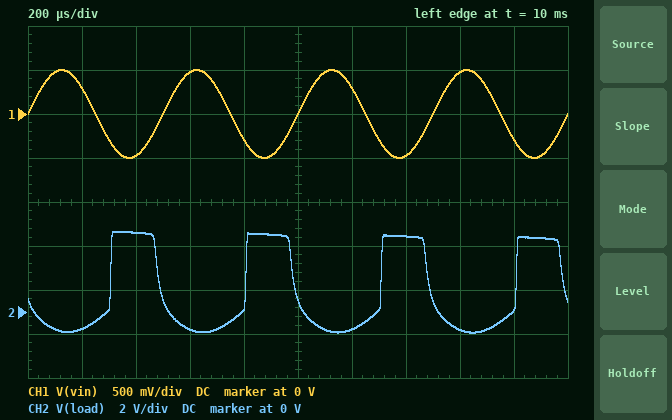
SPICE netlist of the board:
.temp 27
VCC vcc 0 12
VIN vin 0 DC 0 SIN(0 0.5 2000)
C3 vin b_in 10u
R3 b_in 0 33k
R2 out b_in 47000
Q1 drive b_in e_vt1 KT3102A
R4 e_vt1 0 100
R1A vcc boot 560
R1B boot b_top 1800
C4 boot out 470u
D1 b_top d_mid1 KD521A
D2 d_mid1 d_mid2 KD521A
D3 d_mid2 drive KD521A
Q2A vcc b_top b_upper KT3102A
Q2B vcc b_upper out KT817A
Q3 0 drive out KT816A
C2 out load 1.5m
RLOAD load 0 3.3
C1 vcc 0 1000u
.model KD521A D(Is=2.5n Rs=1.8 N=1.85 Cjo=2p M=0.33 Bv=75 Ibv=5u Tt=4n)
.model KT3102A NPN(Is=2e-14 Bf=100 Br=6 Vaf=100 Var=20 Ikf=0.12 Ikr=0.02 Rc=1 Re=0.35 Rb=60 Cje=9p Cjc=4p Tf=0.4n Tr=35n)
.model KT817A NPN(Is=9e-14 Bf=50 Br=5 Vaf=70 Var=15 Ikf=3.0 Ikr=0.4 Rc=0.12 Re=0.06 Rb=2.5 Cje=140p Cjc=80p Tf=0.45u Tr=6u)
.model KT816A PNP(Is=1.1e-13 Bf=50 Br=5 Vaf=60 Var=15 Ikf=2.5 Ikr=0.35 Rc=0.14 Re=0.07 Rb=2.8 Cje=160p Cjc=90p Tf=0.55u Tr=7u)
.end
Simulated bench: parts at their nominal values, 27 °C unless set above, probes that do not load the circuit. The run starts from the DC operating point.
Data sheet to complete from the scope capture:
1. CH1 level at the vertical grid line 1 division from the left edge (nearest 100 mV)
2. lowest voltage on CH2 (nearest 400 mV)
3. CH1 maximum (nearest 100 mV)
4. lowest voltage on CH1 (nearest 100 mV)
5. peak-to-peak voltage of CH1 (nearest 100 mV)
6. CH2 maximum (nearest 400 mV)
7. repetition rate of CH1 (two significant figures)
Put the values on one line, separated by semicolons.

300 mV; -800 mV; 500 mV; -500 mV; 1.0 V; 3.6 V; 2.0 kHz
